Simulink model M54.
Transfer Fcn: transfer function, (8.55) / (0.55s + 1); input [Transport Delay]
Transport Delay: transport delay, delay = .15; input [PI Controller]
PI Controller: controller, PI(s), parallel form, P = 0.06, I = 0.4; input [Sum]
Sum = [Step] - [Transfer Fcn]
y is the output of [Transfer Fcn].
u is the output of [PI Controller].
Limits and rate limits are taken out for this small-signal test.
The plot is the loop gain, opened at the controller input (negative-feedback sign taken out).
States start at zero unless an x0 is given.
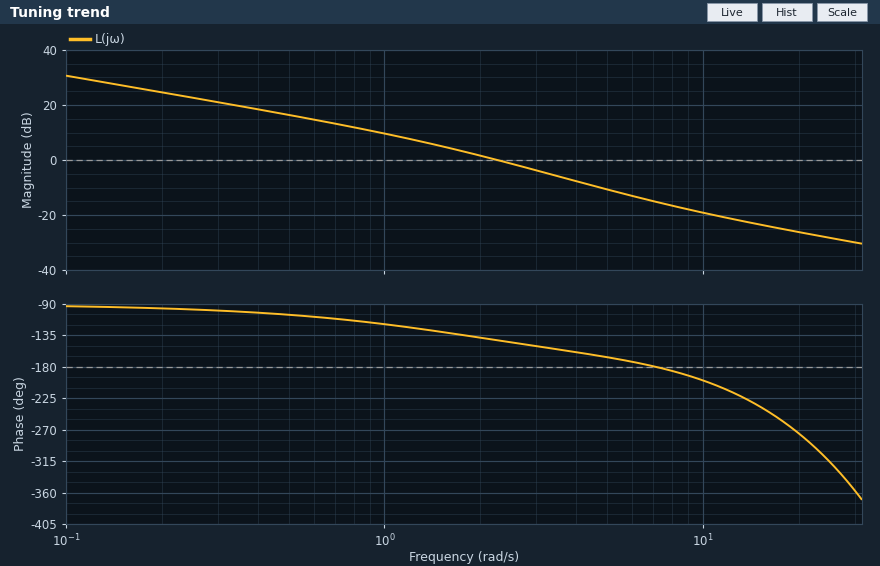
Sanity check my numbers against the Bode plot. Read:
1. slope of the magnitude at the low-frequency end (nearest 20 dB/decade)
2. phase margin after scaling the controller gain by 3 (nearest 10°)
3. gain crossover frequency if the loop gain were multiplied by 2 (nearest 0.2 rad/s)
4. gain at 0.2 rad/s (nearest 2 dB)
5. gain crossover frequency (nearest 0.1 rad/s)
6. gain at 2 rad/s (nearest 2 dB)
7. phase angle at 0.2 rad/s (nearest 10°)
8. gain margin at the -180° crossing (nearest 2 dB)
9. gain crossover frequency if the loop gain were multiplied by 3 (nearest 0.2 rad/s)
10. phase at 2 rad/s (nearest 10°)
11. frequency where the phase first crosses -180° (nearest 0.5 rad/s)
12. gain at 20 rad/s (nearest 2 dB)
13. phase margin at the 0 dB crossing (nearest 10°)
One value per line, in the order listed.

-20 dB/decade
20°
3.6 rad/s
24 dB
2.3 rad/s
2 dB
-100°
16 dB
4.6 rad/s
-140°
7.0 rad/s
-26 dB
40°
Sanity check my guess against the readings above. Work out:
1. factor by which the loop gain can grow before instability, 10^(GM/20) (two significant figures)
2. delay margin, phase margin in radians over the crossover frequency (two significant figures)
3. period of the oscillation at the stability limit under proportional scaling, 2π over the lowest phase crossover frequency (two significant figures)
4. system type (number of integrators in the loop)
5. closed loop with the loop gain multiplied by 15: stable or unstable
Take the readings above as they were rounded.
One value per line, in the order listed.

6.3
0.30 s
0.90 s
1
unstable
